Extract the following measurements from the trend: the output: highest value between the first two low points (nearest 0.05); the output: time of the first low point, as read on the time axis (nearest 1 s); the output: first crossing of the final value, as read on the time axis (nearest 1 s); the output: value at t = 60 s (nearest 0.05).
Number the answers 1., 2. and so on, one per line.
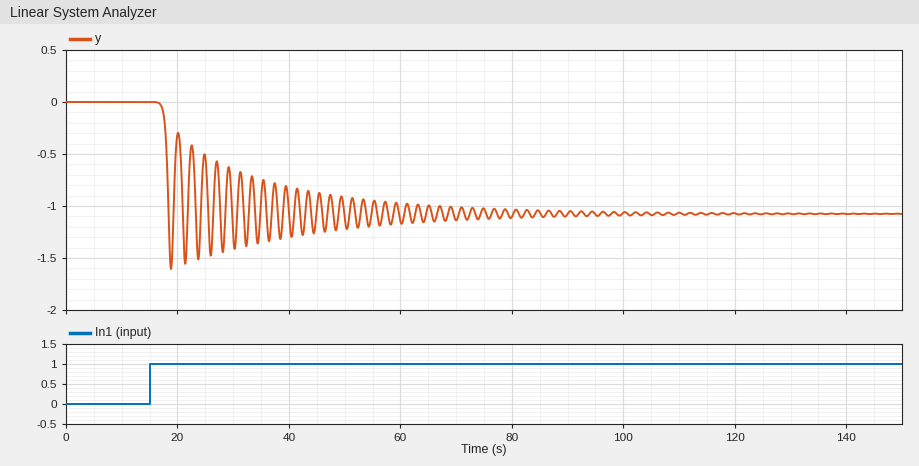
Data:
1. -0.30
2. 19 s
3. 18 s
4. -1.15
